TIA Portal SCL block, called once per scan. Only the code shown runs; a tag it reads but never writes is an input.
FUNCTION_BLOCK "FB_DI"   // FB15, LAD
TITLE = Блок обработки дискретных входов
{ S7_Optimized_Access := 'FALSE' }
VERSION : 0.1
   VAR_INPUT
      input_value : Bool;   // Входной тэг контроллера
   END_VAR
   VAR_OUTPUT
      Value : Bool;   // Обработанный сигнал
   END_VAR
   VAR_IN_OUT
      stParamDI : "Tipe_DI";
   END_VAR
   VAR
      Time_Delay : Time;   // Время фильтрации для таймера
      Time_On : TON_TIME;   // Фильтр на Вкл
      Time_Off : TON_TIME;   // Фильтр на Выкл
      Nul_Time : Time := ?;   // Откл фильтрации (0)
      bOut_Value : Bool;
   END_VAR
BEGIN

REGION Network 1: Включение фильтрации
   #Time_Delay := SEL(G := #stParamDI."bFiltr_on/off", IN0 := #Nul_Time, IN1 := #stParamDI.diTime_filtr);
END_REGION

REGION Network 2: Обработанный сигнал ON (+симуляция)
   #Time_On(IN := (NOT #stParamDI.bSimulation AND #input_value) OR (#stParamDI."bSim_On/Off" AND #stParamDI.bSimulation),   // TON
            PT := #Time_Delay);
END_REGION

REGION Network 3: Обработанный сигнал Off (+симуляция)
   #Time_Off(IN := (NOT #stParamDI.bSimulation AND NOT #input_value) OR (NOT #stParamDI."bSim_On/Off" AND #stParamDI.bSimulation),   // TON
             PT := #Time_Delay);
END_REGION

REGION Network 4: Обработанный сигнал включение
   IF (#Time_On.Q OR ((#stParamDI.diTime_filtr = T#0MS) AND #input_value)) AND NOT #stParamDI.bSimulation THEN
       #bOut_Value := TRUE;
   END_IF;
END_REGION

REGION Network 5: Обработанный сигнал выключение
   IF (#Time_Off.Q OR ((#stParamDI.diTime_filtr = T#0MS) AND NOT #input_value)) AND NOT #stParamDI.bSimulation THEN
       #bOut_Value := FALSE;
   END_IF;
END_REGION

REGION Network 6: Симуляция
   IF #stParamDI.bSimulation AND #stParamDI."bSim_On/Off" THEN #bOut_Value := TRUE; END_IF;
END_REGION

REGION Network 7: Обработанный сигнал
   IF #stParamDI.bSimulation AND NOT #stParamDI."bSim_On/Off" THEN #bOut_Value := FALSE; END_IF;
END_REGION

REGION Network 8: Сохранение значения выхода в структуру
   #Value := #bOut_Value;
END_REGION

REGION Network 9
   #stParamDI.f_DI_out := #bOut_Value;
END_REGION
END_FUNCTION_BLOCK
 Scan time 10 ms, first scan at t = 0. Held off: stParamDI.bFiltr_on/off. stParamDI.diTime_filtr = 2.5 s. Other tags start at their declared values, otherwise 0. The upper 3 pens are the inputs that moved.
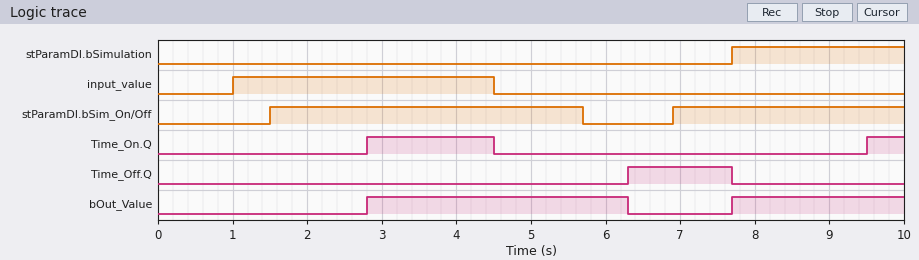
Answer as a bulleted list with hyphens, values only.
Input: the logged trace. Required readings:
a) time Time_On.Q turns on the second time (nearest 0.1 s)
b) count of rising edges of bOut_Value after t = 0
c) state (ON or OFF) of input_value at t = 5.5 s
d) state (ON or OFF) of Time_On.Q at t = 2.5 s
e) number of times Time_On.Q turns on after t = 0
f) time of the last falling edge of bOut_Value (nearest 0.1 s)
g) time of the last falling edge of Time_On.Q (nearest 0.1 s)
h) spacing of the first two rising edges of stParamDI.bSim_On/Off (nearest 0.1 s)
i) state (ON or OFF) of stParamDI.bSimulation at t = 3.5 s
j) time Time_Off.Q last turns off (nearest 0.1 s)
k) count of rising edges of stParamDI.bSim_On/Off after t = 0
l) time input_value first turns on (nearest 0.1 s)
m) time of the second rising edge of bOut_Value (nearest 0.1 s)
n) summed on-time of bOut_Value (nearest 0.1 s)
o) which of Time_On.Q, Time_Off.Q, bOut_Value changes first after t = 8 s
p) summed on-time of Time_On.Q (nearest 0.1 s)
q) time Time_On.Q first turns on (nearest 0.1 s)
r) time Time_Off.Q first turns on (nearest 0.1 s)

- 9.5 s
- 2
- OFF
- OFF
- 2
- 6.3 s
- 4.5 s
- 5.4 s
- OFF
- 7.7 s
- 2
- 1.0 s
- 7.7 s
- 5.8 s
- Time_On.Q
- 2.2 s
- 2.8 s
- 6.3 s
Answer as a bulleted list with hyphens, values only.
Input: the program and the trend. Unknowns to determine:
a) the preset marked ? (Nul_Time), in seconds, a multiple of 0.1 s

- 1.8 s
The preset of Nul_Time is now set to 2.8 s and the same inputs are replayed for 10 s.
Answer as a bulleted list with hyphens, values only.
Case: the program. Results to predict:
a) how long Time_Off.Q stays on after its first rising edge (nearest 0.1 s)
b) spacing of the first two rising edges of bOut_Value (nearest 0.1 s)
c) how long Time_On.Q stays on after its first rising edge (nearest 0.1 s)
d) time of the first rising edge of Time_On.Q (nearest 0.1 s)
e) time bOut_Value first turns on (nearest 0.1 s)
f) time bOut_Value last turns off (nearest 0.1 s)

- 0.4 s
- 3.9 s
- 0.7 s
- 3.8 s
- 3.8 s
- 7.3 s
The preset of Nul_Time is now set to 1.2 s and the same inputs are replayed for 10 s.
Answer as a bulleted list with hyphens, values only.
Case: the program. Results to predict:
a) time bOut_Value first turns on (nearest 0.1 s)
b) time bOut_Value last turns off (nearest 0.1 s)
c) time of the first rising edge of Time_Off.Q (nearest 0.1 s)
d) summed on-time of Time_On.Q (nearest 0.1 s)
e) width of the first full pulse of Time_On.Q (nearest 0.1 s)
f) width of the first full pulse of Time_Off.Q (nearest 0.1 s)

- 2.2 s
- 5.7 s
- 5.7 s
- 3.4 s
- 2.3 s
- 2.0 s
